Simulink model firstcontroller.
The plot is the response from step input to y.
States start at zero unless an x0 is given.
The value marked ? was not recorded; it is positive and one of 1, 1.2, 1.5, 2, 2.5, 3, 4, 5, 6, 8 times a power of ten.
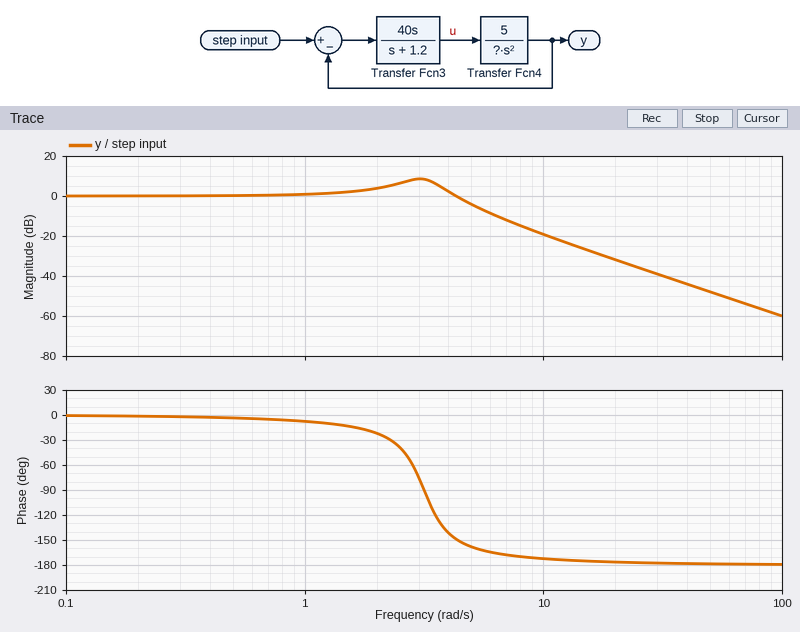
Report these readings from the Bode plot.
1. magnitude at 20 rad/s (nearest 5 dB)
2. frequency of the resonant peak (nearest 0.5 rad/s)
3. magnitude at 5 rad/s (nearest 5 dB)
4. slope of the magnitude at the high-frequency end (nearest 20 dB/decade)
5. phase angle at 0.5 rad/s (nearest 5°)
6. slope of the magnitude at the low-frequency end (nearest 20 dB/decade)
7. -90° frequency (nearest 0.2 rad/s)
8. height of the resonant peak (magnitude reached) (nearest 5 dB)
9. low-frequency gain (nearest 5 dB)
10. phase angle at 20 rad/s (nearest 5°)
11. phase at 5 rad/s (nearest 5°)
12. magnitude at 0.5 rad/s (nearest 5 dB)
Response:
-30 dB
3.0 rad/s
-5 dB
-40 dB/decade
-5°
0 dB/decade
3.2 rad/s
10 dB
0 dB
-175°
-160°
0 dB
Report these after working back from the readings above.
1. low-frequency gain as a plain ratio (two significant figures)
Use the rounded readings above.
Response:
1.0
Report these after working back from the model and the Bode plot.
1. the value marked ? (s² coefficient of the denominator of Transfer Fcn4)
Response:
20
